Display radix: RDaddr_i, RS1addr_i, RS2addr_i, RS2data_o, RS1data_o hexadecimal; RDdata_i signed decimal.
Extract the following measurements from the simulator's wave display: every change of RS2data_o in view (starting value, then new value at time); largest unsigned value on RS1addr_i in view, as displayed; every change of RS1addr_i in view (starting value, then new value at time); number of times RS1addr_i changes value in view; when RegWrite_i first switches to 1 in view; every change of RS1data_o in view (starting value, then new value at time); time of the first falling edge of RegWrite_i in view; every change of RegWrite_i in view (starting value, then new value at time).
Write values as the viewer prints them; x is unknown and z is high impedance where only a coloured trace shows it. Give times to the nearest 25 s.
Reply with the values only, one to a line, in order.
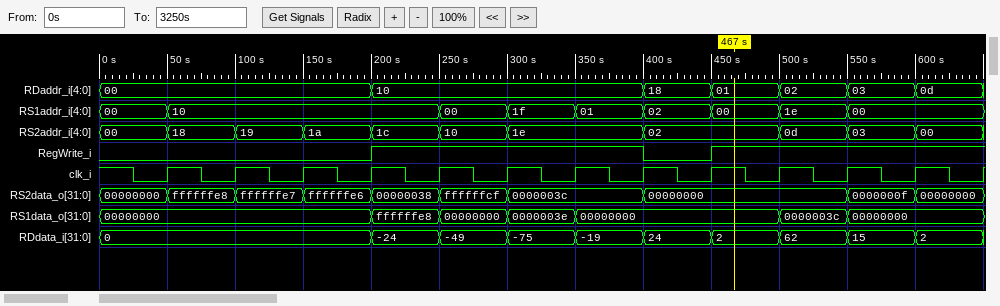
00000000, ffffffe8 at 50 s, ffffffe7 at 100 s, ffffffe6 at 150 s, 00000038 at 200 s, ffffffcf at 250 s, 0000003c at 300 s, 00000000 at 400 s, 0000000f at 550 s, 00000000 at 600 s
1f
00, 10 at 50 s, 00 at 250 s, 1f at 300 s, 01 at 350 s, 02 at 400 s, 00 at 450 s, 1e at 500 s, 00 at 550 s
8
200 s
00000000, ffffffe8 at 200 s, 00000000 at 250 s, 0000003e at 300 s, 00000000 at 350 s, 0000003c at 500 s, 00000000 at 550 s
400 s
0, 1 at 200 s, 0 at 400 s, 1 at 450 s
